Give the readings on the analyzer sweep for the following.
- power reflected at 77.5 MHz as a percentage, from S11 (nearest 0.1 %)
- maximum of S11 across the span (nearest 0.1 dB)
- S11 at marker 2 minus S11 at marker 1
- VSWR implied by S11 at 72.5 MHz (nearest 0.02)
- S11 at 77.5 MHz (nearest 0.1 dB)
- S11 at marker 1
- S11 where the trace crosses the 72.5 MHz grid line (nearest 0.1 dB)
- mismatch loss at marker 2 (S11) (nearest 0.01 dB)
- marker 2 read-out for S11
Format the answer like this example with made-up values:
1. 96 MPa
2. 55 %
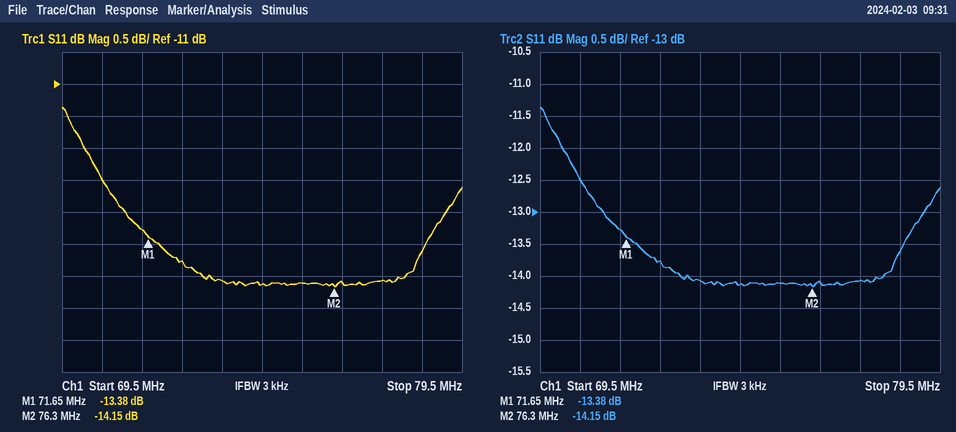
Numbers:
1. 3.9 %
2. -11.4 dB
3. -0.77 dB
4. 1.52
5. -14.1 dB
6. -13.38 dB
7. -13.8 dB
8. 0.17 dB
9. -14.15 dB
